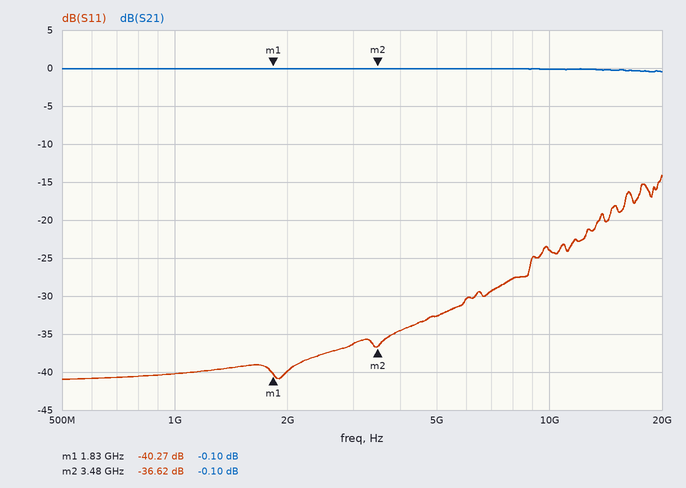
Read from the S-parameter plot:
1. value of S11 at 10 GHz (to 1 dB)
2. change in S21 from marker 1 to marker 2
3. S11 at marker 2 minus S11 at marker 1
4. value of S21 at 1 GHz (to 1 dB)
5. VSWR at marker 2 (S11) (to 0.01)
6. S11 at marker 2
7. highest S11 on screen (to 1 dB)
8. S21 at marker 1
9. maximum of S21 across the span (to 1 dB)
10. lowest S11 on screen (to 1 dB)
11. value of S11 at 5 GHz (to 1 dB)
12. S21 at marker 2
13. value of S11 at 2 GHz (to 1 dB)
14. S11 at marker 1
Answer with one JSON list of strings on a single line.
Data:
["-24 dB", "0.00 dB", "3.65 dB", "0 dB", "1.03", "-36.62 dB", "-14 dB", "-0.10 dB", "0 dB", "-41 dB", "-33 dB", "-0.10 dB", "-40 dB", "-40.27 dB"]
